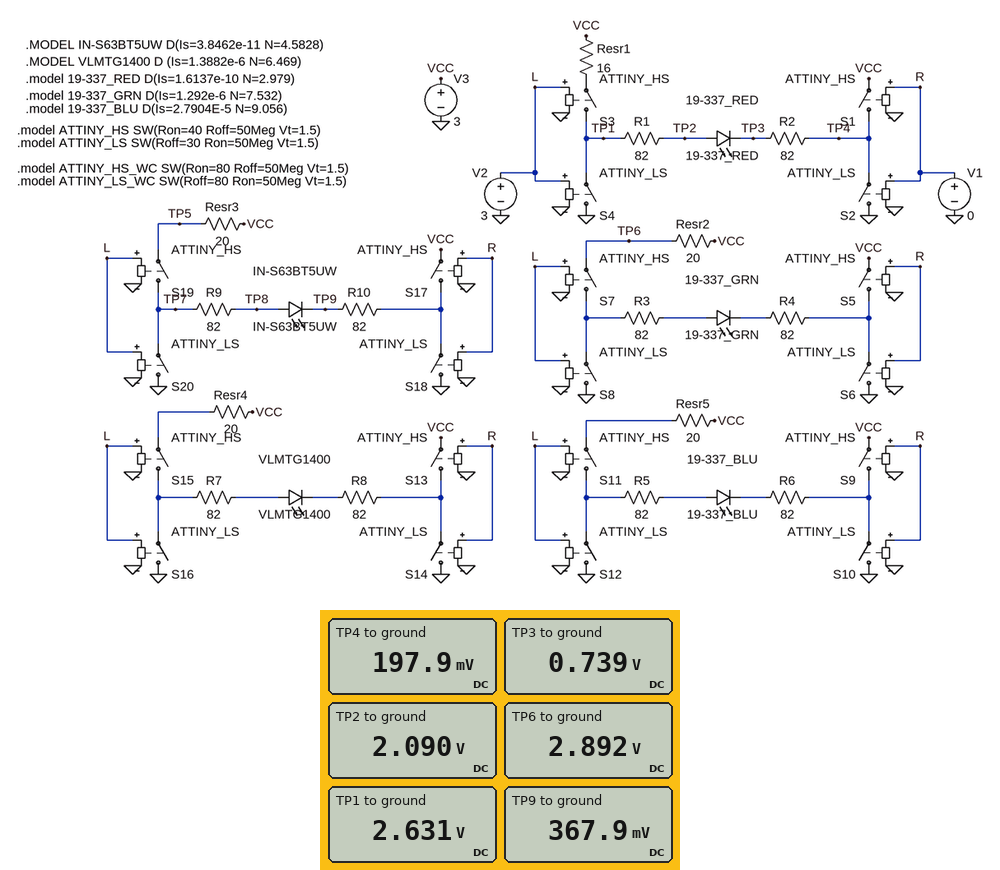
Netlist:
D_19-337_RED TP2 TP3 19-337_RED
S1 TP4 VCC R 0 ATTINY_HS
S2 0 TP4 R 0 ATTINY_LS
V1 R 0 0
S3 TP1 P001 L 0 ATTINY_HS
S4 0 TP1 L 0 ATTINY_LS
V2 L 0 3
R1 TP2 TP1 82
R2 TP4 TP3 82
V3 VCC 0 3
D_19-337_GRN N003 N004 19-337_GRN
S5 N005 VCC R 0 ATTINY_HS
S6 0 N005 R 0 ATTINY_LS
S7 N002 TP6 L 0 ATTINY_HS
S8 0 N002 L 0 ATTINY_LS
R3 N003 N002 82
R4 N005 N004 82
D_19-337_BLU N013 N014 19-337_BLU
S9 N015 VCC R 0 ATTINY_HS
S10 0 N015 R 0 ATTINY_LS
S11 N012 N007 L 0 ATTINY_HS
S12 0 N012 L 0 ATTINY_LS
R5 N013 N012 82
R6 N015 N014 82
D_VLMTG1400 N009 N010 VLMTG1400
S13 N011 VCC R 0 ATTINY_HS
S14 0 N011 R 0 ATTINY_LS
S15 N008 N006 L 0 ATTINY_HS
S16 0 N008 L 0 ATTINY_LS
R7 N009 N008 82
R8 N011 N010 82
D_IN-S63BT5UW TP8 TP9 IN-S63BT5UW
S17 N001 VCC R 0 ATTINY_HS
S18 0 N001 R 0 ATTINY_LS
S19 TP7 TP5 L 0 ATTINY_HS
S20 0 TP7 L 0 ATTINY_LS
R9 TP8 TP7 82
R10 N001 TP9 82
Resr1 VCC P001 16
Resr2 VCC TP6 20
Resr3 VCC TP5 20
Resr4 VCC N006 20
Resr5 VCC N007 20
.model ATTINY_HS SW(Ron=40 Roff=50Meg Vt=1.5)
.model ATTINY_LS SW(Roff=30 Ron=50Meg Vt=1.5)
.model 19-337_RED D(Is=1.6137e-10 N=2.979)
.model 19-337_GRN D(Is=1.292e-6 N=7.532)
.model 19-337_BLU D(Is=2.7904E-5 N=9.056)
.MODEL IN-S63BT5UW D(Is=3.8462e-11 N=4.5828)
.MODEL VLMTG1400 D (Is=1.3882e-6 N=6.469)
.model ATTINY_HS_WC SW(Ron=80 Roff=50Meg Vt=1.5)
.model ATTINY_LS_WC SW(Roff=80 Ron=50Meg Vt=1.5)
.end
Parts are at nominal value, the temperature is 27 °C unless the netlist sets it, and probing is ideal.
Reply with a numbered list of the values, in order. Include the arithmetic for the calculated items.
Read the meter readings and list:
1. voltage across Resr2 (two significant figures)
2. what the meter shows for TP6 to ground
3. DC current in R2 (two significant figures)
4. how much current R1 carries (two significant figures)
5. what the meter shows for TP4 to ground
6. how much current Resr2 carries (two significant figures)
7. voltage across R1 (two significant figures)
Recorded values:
1. 3 V - 2.892 V = 110 mV
2. 2.892 V
3. (739 mV - 197.9 mV) / 82 Ω = 6.6 mA
4. (2.631 V - 2.09 V) / 82 Ω = 6.6 mA
5. 197.9 mV
6. (3 V - 2.892 V) / 20 Ω = 5.4 mA
7. 2.631 V - 2.09 V = 540 mV
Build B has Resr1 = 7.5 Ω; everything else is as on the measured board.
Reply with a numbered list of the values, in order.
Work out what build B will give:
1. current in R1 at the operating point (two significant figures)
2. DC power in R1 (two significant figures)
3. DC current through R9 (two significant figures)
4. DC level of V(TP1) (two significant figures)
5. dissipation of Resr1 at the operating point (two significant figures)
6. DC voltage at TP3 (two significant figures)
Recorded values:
1. 6.8 mA
2. 3.8 mW
3. 3.3 mA
4. 2.7 V
5. 350 µW
6. 760 mV
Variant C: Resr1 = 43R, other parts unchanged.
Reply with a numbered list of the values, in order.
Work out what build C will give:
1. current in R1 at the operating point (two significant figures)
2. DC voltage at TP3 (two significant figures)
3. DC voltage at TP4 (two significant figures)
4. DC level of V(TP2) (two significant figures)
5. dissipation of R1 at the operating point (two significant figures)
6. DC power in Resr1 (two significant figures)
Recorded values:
1. 6.0 mA
2. 670 mV
3. 180 mV
4. 2.0 V
5. 2.9 mW
6. 1.5 mW
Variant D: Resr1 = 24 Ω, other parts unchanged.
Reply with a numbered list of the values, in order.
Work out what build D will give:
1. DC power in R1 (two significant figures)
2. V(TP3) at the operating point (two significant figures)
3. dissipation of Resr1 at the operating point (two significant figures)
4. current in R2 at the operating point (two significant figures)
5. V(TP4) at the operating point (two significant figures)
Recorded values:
1. 3.4 mW
2. 720 mV
3. 980 µW
4. 6.4 mA
5. 190 mV
